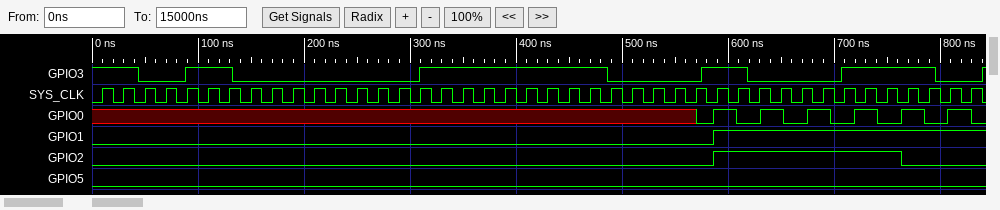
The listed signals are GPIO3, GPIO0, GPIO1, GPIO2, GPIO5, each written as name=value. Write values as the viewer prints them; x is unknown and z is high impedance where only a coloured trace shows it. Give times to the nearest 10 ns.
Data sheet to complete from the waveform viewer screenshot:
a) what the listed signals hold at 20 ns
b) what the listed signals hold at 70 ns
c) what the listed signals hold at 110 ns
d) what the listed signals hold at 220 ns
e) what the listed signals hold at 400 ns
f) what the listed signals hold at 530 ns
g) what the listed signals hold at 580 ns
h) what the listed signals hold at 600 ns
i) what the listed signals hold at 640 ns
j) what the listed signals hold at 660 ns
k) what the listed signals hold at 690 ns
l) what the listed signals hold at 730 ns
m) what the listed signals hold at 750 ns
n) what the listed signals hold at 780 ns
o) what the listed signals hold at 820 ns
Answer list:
GPIO3=1, GPIO0=x, GPIO1=0, GPIO2=0, GPIO5=0
GPIO3=0, GPIO0=x, GPIO1=0, GPIO2=0, GPIO5=0
GPIO3=1, GPIO0=x, GPIO1=0, GPIO2=0, GPIO5=0
GPIO3=0, GPIO0=x, GPIO1=0, GPIO2=0, GPIO5=0
GPIO3=1, GPIO0=x, GPIO1=0, GPIO2=0, GPIO5=0
GPIO3=0, GPIO0=x, GPIO1=0, GPIO2=0, GPIO5=0
GPIO3=1, GPIO0=0, GPIO1=0, GPIO2=0, GPIO5=0
GPIO3=1, GPIO0=1, GPIO1=1, GPIO2=1, GPIO5=0
GPIO3=0, GPIO0=1, GPIO1=1, GPIO2=1, GPIO5=0
GPIO3=0, GPIO0=0, GPIO1=1, GPIO2=1, GPIO5=0
GPIO3=0, GPIO0=1, GPIO1=1, GPIO2=1, GPIO5=0
GPIO3=1, GPIO0=1, GPIO1=1, GPIO2=1, GPIO5=0
GPIO3=1, GPIO0=0, GPIO1=1, GPIO2=1, GPIO5=0
GPIO3=1, GPIO0=1, GPIO1=1, GPIO2=0, GPIO5=0
GPIO3=0, GPIO0=1, GPIO1=1, GPIO2=0, GPIO5=0
